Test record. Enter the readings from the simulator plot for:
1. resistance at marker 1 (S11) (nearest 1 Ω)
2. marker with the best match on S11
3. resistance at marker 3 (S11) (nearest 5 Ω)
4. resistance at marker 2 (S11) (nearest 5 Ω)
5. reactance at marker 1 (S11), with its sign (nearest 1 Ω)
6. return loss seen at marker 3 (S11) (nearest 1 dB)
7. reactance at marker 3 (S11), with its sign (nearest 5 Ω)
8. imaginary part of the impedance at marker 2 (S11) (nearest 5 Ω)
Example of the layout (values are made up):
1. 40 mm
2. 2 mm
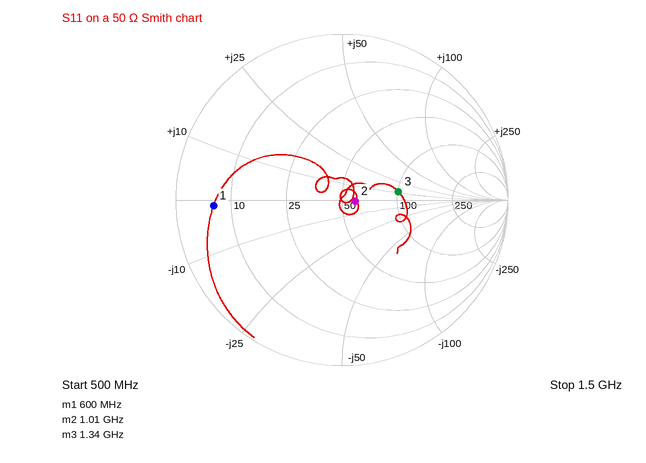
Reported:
1. 6 Ω
2. marker 2
3. 100 Ω
4. 60 Ω
5. -1 Ω
6. 9 dB
7. +10 Ω
8. 0 Ω
